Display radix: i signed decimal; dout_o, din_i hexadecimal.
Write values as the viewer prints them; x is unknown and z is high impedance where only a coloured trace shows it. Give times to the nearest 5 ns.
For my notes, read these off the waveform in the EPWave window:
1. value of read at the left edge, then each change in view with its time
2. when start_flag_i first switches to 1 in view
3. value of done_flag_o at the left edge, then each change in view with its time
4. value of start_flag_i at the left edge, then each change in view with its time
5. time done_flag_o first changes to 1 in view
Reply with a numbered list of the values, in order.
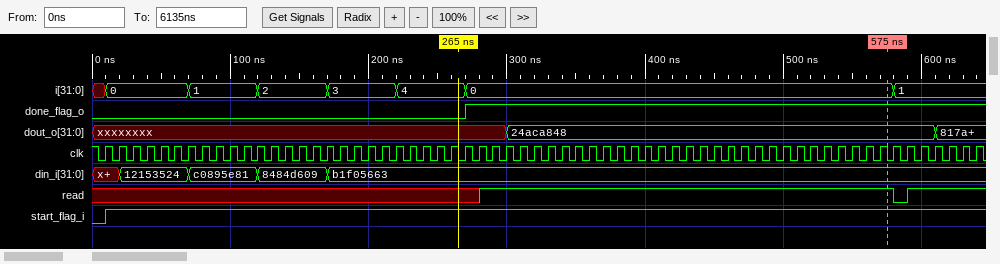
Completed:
1. x, 1 at 280 ns, 0 at 580 ns, 1 at 590 ns
2. 10 ns
3. 0, 1 at 270 ns
4. 0, 1 at 10 ns
5. 270 ns
